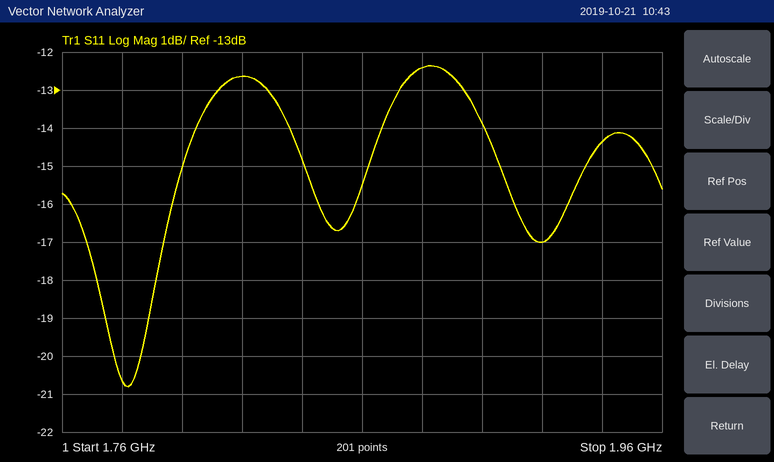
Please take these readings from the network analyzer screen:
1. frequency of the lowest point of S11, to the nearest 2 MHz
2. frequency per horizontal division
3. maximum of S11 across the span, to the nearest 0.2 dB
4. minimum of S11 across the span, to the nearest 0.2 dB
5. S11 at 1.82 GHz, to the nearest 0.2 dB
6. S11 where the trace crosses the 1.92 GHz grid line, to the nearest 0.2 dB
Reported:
1.782 GHz
20 MHz
-12.4 dB
-20.8 dB
-12.6 dB
-17.0 dB
